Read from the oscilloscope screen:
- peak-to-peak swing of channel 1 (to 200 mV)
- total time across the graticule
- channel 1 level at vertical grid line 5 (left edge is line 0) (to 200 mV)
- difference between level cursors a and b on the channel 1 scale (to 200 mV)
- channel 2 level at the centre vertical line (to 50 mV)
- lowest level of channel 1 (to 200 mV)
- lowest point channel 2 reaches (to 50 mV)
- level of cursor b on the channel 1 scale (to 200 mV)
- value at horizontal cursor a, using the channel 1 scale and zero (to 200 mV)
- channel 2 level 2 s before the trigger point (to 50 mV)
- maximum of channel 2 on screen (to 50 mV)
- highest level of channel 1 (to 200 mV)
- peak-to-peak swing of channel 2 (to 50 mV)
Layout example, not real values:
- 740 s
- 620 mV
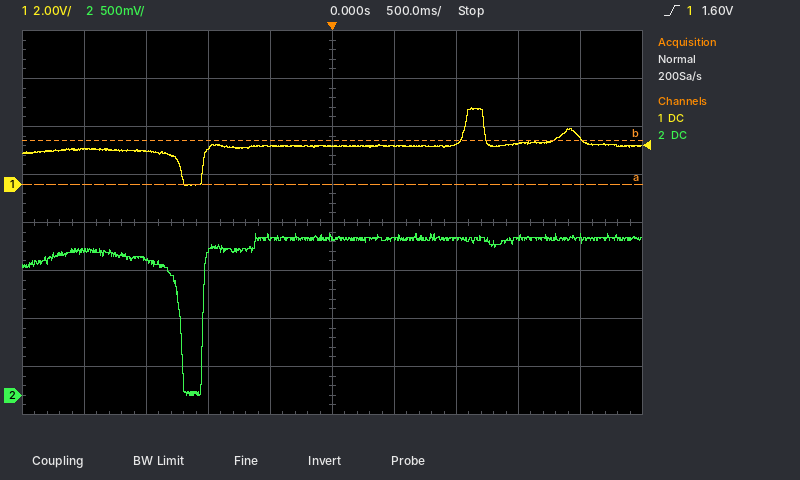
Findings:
- 3.2 V
- 5 s
- 1.6 V
- 1.8 V
- 1.65 V
- 0.0 V
- 0 mV
- 1.8 V
- 0.0 V
- 1.50 V
- 1.70 V
- 3.2 V
- 1.70 V
